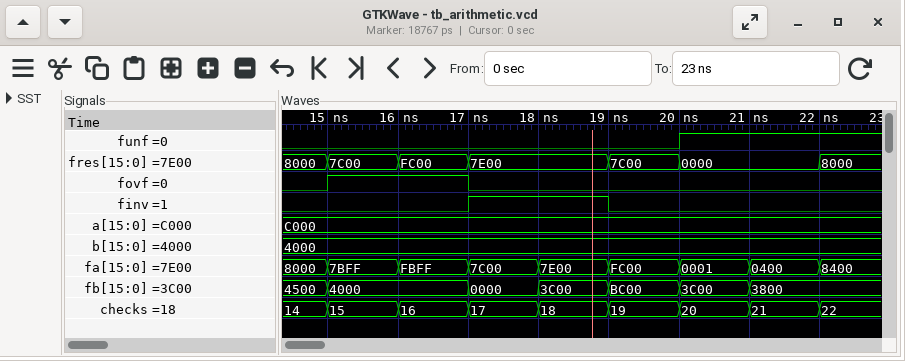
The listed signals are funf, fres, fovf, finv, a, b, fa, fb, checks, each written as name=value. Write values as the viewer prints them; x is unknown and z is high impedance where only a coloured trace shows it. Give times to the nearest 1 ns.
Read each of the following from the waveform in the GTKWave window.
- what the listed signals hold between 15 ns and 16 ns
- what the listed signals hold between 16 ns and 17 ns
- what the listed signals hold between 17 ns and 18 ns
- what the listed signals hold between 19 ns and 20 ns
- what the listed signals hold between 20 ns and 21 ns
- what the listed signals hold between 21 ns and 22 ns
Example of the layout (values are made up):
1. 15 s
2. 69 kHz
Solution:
1. funf=0, fres=7C00, fovf=1, finv=0, a=C000, b=4000, fa=7BFF, fb=4000, checks=15
2. funf=0, fres=FC00, fovf=1, finv=0, a=C000, b=4000, fa=FBFF, fb=4000, checks=16
3. funf=0, fres=7E00, fovf=0, finv=1, a=C000, b=4000, fa=7C00, fb=0000, checks=17
4. funf=0, fres=7C00, fovf=0, finv=0, a=C000, b=4000, fa=FC00, fb=BC00, checks=19
5. funf=1, fres=0000, fovf=0, finv=0, a=C000, b=4000, fa=0001, fb=3C00, checks=20
6. funf=1, fres=0000, fovf=0, finv=0, a=C000, b=4000, fa=0400, fb=3800, checks=21
